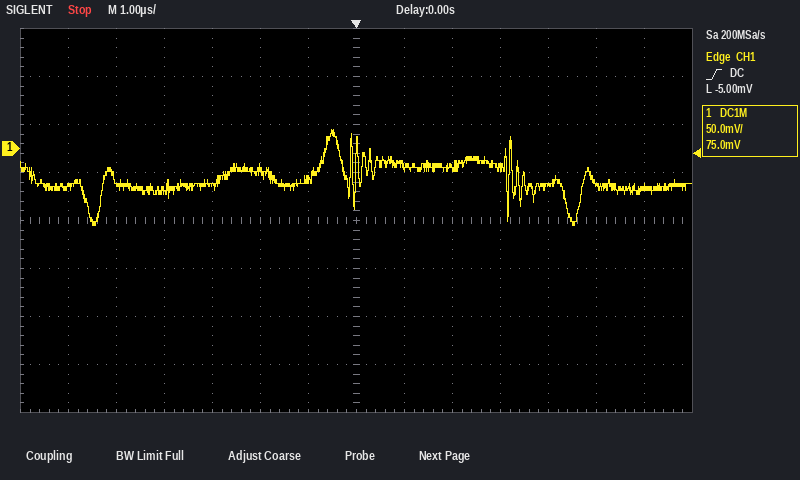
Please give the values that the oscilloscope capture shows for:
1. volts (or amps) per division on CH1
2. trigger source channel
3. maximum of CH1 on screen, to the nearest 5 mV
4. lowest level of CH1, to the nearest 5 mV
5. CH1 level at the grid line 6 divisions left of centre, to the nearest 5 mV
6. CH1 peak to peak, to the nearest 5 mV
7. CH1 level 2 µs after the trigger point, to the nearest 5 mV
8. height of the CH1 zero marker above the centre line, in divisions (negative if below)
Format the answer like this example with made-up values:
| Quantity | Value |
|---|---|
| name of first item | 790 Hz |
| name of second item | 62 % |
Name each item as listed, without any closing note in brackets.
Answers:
| Quantity | Value |
|---|---|
| volts (or amps) per division on CH1 | 50 mV |
| trigger source channel | CH1 |
| maximum of CH1 on screen, to the nearest 5 mV | 20 mV |
| lowest level of CH1, to the nearest 5 mV | -80 mV |
| CH1 level at the grid line 6 divisions left of centre, to the nearest 5 mV | -40 mV |
| CH1 peak to peak, to the nearest 5 mV | 100 mV |
| CH1 level 2 µs after the trigger point, to the nearest 5 mV | -20 mV |
| height of the CH1 zero marker above the centre line, in divisions | +1.5 div |
